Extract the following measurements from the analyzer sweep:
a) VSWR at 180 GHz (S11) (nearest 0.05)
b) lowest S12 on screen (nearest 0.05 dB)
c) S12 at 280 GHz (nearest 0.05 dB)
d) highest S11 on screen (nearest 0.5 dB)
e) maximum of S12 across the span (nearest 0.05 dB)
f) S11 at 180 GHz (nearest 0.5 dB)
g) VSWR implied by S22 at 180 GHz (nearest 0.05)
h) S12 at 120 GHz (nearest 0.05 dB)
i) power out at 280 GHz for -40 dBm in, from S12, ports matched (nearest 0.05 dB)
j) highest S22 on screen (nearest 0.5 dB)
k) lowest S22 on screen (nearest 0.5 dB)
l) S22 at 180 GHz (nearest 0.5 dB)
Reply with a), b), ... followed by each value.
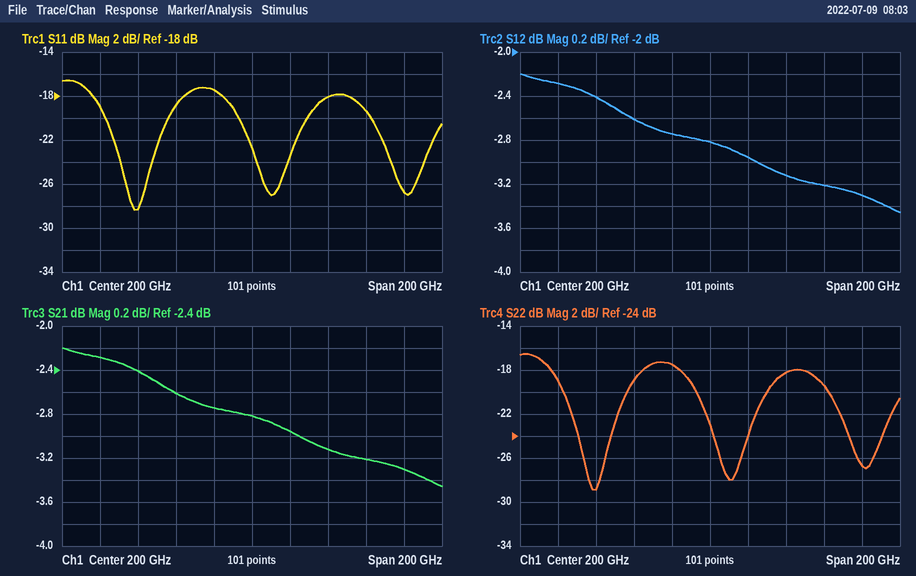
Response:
a) 1.30
b) -3.45 dB
c) -3.30 dB
d) -16.5 dB
e) -2.20 dB
f) -17.5 dB
g) 1.30
h) -2.30 dB
i) -43.30 dBm
j) -16.5 dB
k) -29.0 dB
l) -17.5 dB
